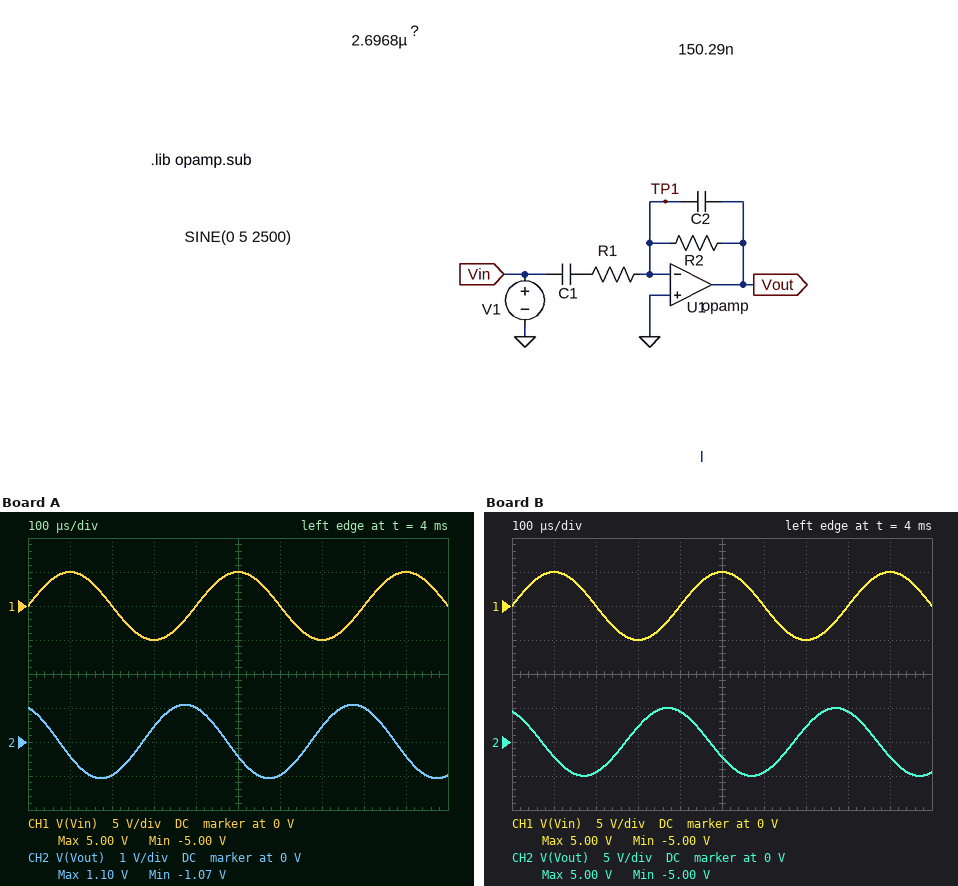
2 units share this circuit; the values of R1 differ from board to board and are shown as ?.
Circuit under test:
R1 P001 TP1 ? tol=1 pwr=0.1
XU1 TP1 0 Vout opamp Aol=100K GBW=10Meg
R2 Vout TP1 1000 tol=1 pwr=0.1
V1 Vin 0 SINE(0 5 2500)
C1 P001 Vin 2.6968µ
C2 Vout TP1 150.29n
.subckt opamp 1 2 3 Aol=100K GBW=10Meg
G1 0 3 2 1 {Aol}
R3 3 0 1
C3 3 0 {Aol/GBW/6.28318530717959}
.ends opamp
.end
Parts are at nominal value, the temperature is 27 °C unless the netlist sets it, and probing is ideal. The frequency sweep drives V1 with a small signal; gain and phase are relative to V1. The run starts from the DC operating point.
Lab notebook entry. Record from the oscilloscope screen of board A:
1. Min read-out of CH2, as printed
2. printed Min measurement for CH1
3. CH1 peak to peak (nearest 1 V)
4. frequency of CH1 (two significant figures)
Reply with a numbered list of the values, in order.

1. -1.07 V
2. -5.00 V
3. 10 V
4. 2.5 kHz
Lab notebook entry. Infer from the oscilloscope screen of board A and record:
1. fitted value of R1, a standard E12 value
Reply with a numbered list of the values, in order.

1. 1.8 kΩ
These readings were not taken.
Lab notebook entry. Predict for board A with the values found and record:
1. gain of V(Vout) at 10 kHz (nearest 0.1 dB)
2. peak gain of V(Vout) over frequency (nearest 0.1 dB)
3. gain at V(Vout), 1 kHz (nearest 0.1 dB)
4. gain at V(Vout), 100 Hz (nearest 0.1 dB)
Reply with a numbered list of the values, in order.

1. -24.7 dB
2. -5.4 dB
3. -7.9 dB
4. -5.6 dB
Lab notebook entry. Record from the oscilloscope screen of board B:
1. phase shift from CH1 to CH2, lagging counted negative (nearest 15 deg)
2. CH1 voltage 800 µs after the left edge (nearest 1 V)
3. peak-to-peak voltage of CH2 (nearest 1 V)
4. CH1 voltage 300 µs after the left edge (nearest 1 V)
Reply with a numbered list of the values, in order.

1. 120 deg
2. 0 V
3. 10 V
4. -5 V
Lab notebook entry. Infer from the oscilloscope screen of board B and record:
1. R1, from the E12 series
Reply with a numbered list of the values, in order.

1. 390 Ω
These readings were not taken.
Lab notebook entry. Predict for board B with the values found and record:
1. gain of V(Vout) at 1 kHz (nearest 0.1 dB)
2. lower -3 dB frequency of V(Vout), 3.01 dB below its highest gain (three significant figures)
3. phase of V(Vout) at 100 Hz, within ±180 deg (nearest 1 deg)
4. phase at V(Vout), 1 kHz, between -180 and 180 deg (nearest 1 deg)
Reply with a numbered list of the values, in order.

1. 5.3 dB
2. 120 Hz
3. -129 deg
4. 145 deg
